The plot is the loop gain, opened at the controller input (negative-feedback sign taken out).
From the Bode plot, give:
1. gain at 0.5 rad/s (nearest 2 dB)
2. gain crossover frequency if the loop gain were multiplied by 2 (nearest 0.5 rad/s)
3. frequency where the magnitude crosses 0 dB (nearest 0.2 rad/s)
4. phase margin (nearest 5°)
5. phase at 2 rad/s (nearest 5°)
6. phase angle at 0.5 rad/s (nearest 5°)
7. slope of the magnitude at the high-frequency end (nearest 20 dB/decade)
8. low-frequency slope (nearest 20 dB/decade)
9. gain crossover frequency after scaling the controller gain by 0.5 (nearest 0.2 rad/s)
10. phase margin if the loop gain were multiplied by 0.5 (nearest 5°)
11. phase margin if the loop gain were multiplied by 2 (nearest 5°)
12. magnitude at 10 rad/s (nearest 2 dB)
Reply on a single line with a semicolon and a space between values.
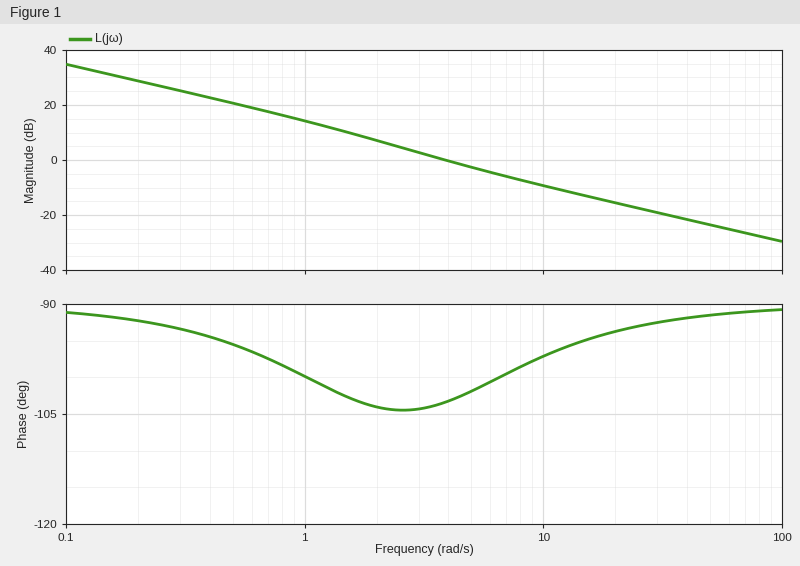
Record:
20 dB; 7.0 rad/s; 3.8 rad/s; 75°; -105°; -95°; -20 dB/decade; -20 dB/decade; 2.2 rad/s; 75°; 80°; -10 dB
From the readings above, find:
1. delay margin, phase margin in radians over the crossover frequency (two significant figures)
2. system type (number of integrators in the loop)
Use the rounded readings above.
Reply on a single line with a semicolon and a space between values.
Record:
0.34 s; 1
